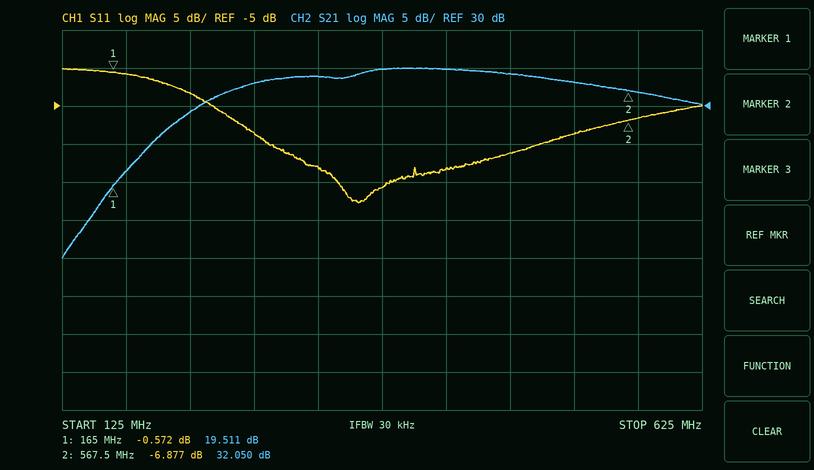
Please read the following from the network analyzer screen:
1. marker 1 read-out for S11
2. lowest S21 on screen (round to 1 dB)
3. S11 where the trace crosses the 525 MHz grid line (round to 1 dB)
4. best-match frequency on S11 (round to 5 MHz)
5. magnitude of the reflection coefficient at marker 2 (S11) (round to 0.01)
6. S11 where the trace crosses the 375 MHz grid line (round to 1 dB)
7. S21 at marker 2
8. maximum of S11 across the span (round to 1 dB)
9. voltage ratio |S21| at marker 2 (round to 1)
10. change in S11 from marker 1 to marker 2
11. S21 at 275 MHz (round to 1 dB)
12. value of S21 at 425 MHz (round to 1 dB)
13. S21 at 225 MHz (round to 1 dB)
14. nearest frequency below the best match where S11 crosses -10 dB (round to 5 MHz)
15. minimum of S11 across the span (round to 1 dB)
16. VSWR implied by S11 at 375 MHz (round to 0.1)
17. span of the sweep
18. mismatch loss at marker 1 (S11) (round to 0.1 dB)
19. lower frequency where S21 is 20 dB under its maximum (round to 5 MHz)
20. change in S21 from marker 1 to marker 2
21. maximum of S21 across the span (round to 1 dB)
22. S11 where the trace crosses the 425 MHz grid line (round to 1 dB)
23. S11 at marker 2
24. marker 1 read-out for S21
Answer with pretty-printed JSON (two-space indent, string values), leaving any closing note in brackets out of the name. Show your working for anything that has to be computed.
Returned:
{
  "marker 1 read-out for S11": "-0.572 dB",
  "lowest S21 on screen": "10 dB",
  "S11 where the trace crosses the 525 MHz grid line": "-9 dB",
  "best-match frequency on S11": "355 MHz",
  "magnitude of the reflection coefficient at marker 2 (S11)": "10^(-6.877/20) ≈ 0.45",
  "S11 where the trace crosses the 375 MHz grid line": "-16 dB",
  "S21 at marker 2": "32.050 dB",
  "maximum of S11 across the span": "0 dB",
  "voltage ratio |S21| at marker 2": "10^(32.05/20) ≈ 40",
  "change in S11 from marker 1 to marker 2": "-6.877 − (-0.572) = -6.305 dB",
  "S21 at 275 MHz": "33 dB",
  "value of S21 at 425 MHz": "35 dB",
  "S21 at 225 MHz": "29 dB",
  "nearest frequency below the best match where S11 crosses -10 dB": "285 MHz",
  "minimum of S11 across the span": "-18 dB",
  "VSWR implied by S11 at 375 MHz": "|Γ| = 10^(-16/20) = 0.1585; VSWR = (1 + 0.1585)/(1 − 0.1585) ≈ 1.4",
  "span of the sweep": "500 MHz",
  "mismatch loss at marker 1 (S11)": "−10 log10(1 − 10^(-0.572/10)) ≈ 9.1 dB",
  "lower frequency where S21 is 20 dB under its maximum": "145 MHz",
  "change in S21 from marker 1 to marker 2": "32.05 − (19.511) = 12.539 dB",
  "maximum of S21 across the span": "35 dB",
  "S11 where the trace crosses the 425 MHz grid line": "-13 dB",
  "S11 at marker 2": "-6.877 dB",
  "marker 1 read-out for S21": "19.511 dB"
}
